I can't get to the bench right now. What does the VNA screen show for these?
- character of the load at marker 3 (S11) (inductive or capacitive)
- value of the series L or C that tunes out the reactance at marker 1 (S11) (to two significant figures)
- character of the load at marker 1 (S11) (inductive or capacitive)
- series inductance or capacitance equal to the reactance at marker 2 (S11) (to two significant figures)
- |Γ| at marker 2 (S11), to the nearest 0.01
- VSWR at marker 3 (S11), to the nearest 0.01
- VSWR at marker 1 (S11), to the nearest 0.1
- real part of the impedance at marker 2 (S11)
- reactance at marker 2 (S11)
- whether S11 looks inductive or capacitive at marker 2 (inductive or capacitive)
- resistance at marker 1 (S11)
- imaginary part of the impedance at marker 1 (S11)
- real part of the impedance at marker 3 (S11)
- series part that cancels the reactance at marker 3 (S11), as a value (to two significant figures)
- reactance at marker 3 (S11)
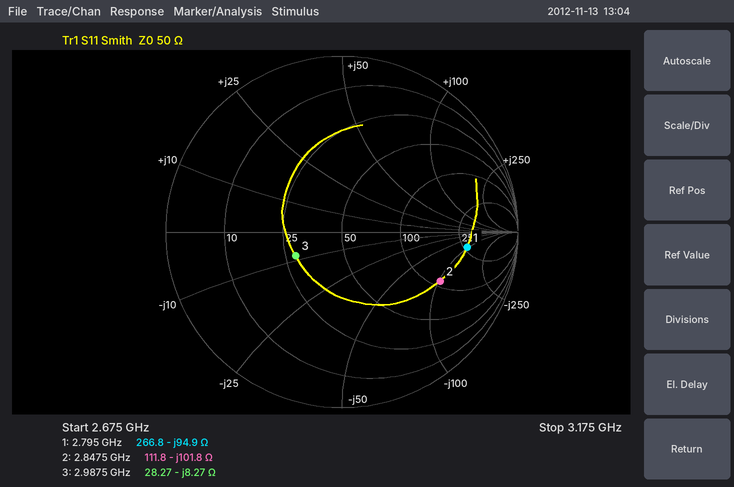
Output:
capacitive
5.4 nH
capacitive
550 fF
0.62
1.84
6.0
111.8 Ω
-101.8 Ω
capacitive
266.8 Ω
-94.9 Ω
28.27 Ω
440 pH
-8.27 Ω
